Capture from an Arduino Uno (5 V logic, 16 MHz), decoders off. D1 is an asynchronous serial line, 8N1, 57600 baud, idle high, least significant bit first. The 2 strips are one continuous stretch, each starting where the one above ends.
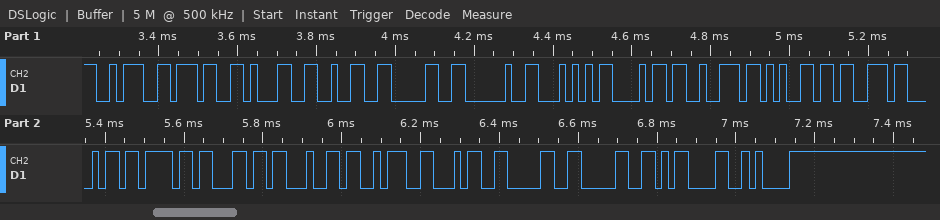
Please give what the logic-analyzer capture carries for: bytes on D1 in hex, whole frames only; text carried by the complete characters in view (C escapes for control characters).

3A 37 31 32 30 20 54 68 72 65 73 68 6F 6C 64 3A 34 30 30 0D 0A
":7120 Threshold:400\r\n"
